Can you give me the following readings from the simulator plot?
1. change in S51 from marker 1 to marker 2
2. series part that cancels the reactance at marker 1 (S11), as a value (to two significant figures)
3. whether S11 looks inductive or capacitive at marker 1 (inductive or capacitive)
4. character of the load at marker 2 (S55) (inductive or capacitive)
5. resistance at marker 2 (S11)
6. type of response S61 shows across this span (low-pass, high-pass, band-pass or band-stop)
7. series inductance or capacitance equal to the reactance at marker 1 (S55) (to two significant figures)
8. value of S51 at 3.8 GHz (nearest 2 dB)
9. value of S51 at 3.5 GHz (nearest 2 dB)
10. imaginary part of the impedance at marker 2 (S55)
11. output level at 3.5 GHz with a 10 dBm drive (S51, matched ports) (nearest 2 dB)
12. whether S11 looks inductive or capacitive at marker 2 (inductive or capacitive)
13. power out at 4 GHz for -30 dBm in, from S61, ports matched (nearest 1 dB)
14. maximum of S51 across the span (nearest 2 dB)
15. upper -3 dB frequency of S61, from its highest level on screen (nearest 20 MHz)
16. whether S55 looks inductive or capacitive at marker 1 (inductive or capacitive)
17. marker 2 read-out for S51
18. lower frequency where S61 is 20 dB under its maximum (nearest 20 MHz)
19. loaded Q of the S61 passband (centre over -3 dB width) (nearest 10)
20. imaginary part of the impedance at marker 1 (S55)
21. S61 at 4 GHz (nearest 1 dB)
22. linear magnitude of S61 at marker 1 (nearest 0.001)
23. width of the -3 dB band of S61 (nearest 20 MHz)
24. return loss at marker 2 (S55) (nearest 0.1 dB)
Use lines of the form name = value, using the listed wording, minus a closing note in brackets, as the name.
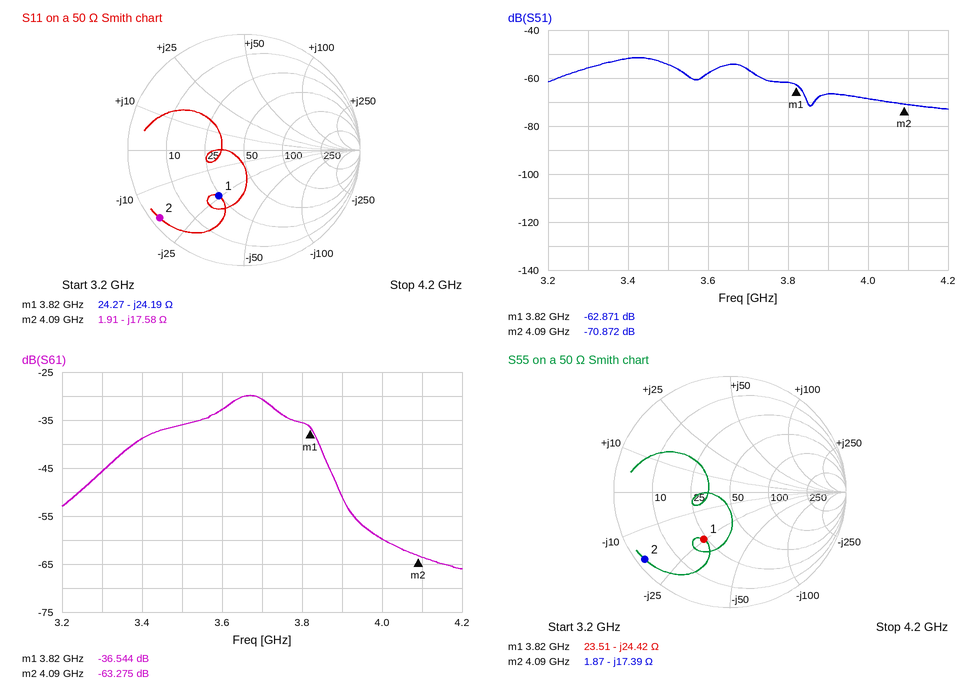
change in S51 from marker 1 to marker 2 = -8.001 dB
series part that cancels the reactance at marker 1 (S11), as a value = 1.0 nH
whether S11 looks inductive or capacitive at marker 1 = capacitive
character of the load at marker 2 (S55) = capacitive
resistance at marker 2 = 1.91 Ω
type of response S61 shows across this span = band-pass
series inductance or capacitance equal to the reactance at marker 1 (S55) = 1.7 pF
value of S51 at 3.8 GHz = -62 dB
value of S51 at 3.5 GHz = -54 dB
imaginary part of the impedance at marker 2 = -17.39 Ω
output level at 3.5 GHz with a 10 dBm drive (S51, matched ports) = -44 dBm
whether S11 looks inductive or capacitive at marker 2 = capacitive
power out at 4 GHz for -30 dBm in, from S61, ports matched = -90 dBm
maximum of S51 across the span = -52 dB
upper -3 dB frequency of S61, from its highest level on screen = 3.74 GHz
whether S55 looks inductive or capacitive at marker 1 = capacitive
marker 2 read-out for S51 = -70.872 dB
lower frequency where S61 is 20 dB under its maximum = 3.24 GHz
loaded Q of the S61 passband (centre over -3 dB width) = 30
imaginary part of the impedance at marker 1 = -24.42 Ω
S61 at 4 GHz = -60 dB
linear magnitude of S61 at marker 1 = 0.015
width of the -3 dB band of S61 = 140 MHz
return loss at marker 2 (S55) = 0.6 dB
